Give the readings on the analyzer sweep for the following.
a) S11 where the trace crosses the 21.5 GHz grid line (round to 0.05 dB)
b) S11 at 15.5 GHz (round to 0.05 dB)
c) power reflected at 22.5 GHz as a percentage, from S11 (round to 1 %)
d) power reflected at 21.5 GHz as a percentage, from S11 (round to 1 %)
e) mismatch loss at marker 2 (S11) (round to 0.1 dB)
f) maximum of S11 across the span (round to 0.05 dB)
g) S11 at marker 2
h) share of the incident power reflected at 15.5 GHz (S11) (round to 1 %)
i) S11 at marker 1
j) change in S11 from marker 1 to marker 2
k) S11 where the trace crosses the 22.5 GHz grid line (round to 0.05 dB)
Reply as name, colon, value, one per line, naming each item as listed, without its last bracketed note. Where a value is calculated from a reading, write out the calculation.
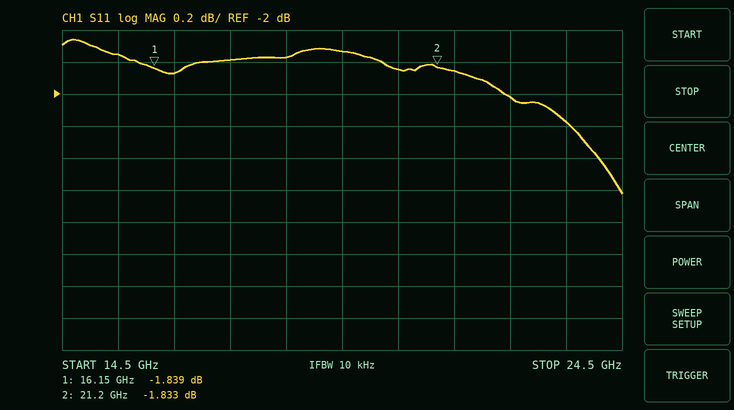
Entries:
S11 where the trace crosses the 21.5 GHz grid line: -1.85 dB
S11 at 15.5 GHz: -1.75 dB
power reflected at 22.5 GHz as a percentage, from S11: 10^(-2/10) ≈ 63 %
power reflected at 21.5 GHz as a percentage, from S11: 10^(-1.85/10) ≈ 65 %
mismatch loss at marker 2 (S11): −10 log10(1 − 10^(-1.833/10)) ≈ 4.6 dB
maximum of S11 across the span: -1.65 dB
S11 at marker 2: -1.833 dB
share of the incident power reflected at 15.5 GHz (S11): 10^(-1.75/10) ≈ 67 %
S11 at marker 1: -1.839 dB
change in S11 from marker 1 to marker 2: -1.833 − (-1.839) = 0.006 dB
S11 where the trace crosses the 22.5 GHz grid line: -2.00 dB
